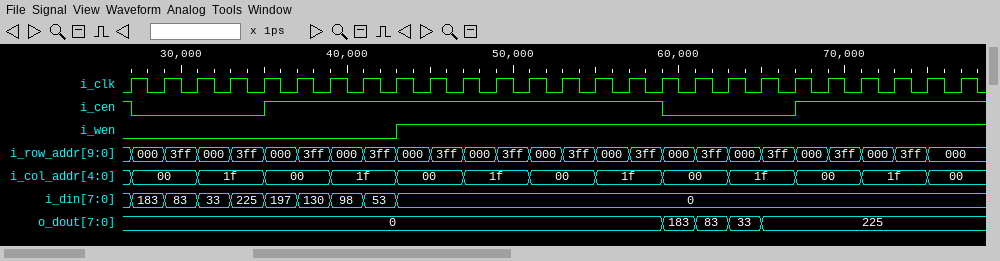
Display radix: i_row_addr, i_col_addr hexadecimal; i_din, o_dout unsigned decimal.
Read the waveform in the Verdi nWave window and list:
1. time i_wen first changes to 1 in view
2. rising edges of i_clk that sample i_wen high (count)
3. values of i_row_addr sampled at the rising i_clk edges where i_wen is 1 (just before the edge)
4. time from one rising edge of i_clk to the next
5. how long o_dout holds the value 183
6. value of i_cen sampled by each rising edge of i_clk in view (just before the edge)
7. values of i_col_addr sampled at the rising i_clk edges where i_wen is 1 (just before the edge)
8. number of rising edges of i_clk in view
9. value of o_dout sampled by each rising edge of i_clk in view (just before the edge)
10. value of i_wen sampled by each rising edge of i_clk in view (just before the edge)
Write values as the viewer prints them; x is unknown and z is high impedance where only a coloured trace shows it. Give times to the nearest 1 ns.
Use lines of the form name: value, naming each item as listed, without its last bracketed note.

time i_wen first changes to 1 in view: 43 ns
rising edges of i_clk that sample i_wen high: 17
values of i_row_addr sampled at the rising i_clk edges where i_wen is 1: 000, 3ff, 000, 3ff, 000, 3ff, 000, 3ff, 000, 3ff, 000, 3ff, 000, 3ff, 000, 3ff, 000
time from one rising edge of i_clk to the next: 2 ns
how long o_dout holds the value 183: 2 ns
value of i_cen sampled by each rising edge of i_clk in view: 1 0 0 0 0 1 1 1 1 1 1 1 1 1 1 1 1 0 0 0 0 1 1 1 1 1
values of i_col_addr sampled at the rising i_clk edges where i_wen is 1: 00, 00, 1f, 1f, 00, 00, 1f, 1f, 00, 00, 1f, 1f, 00, 00, 1f, 1f, 00
number of rising edges of i_clk in view: 26
value of o_dout sampled by each rising edge of i_clk in view: 0, 0, 0, 0, 0, 0, 0, 0, 0, 0, 0, 0, 0, 0, 0, 0, 0, 183, 83, 33, 225, 225, 225, 225, 225, 225
value of i_wen sampled by each rising edge of i_clk in view: 0 0 0 0 0 0 0 0 0 1 1 1 1 1 1 1 1 1 1 1 1 1 1 1 1 1
